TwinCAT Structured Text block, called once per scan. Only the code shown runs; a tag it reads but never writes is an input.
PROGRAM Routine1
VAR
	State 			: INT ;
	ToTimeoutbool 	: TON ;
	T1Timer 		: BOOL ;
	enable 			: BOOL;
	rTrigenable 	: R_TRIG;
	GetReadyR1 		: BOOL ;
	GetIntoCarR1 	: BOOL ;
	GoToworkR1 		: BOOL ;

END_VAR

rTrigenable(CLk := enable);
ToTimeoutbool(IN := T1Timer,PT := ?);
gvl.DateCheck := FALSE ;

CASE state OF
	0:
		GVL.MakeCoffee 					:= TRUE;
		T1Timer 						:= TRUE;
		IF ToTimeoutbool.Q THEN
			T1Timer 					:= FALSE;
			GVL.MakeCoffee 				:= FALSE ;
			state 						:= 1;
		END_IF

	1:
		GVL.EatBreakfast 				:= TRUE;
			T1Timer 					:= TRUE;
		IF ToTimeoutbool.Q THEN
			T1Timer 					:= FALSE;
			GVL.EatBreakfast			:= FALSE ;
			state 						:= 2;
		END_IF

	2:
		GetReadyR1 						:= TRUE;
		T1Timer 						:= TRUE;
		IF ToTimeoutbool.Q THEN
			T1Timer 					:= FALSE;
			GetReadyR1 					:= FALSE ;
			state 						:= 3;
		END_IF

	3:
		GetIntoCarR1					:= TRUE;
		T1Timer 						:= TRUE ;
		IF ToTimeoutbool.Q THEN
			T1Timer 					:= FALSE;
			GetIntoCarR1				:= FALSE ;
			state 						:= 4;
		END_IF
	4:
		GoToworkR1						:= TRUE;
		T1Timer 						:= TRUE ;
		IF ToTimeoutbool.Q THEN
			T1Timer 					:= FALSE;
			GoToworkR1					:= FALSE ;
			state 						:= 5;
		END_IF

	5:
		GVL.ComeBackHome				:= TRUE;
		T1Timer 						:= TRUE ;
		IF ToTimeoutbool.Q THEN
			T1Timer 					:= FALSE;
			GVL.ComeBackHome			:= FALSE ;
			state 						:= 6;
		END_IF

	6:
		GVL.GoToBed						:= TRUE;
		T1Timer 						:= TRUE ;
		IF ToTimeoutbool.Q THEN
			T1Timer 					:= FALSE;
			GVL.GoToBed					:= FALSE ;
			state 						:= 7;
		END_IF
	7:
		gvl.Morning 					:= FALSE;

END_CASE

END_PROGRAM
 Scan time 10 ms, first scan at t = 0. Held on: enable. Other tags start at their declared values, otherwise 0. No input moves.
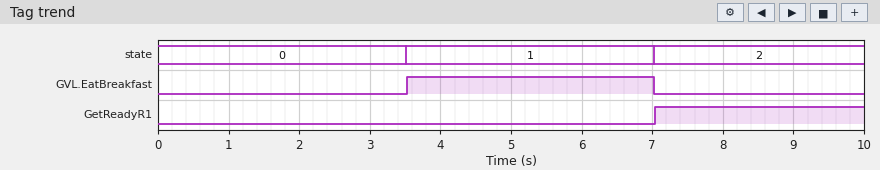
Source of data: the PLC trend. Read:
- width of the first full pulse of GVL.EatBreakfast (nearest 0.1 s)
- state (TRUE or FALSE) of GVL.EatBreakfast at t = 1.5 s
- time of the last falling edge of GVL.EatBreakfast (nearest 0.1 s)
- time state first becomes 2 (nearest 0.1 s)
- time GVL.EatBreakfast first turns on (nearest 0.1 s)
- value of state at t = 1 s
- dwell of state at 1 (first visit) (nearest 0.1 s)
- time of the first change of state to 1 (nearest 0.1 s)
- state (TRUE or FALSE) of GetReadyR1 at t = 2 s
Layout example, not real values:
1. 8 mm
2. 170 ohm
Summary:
1. 3.5 s
2. FALSE
3. 7.0 s
4. 7.0 s
5. 3.5 s
6. 0
7. 3.5 s
8. 3.5 s
9. FALSE
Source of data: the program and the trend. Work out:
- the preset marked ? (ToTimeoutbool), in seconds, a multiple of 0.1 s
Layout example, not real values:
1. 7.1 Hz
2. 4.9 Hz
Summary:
1. 3.5 s
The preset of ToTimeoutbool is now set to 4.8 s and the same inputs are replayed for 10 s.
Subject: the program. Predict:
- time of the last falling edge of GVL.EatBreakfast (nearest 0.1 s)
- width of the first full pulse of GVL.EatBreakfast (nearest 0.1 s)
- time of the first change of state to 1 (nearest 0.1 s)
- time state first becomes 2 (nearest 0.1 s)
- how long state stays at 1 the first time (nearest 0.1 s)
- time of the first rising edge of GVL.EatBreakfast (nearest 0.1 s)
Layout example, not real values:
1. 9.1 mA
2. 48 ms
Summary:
1. 9.6 s
2. 4.8 s
3. 4.8 s
4. 9.6 s
5. 4.8 s
6. 4.8 s
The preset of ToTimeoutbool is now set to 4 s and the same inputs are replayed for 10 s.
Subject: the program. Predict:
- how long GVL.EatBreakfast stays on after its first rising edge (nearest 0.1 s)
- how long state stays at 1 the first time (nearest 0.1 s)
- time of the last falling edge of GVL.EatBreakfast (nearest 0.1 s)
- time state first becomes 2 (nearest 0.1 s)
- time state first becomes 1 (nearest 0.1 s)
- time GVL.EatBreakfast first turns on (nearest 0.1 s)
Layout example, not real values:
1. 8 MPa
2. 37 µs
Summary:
1. 4.0 s
2. 4.0 s
3. 8.0 s
4. 8.0 s
5. 4.0 s
6. 4.0 s
